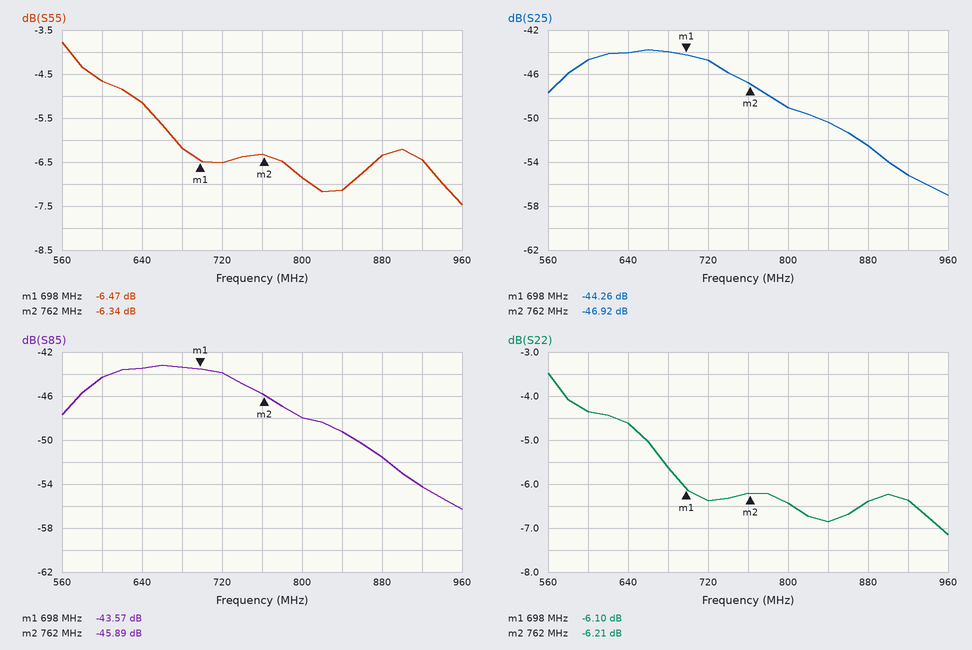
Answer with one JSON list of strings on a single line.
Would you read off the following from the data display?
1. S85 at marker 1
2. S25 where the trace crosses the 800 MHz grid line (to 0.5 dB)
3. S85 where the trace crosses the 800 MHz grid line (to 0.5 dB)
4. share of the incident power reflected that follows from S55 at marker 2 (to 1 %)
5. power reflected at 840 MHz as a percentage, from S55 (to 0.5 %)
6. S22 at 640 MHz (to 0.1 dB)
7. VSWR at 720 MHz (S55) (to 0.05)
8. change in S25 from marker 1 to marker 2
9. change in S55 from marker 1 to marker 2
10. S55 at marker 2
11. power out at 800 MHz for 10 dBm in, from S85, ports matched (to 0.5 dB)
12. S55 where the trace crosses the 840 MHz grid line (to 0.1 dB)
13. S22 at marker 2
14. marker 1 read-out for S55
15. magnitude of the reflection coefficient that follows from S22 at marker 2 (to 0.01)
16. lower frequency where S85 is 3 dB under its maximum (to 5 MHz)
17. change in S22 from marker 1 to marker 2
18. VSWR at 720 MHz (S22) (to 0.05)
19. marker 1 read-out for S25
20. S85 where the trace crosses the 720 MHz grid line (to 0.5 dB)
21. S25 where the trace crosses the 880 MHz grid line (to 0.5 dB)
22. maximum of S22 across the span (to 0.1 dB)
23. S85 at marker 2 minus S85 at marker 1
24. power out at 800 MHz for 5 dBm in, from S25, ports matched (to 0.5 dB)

["-43.57 dB", "-49.0 dB", "-48.0 dB", "23 %", "19.5 %", "-4.6 dB", "2.80", "-2.66 dB", "0.13 dB", "-6.34 dB", "-38.0 dBm", "-7.1 dB", "-6.21 dB", "-6.47 dB", "0.49", "575 MHz", "-0.11 dB", "2.85", "-44.26 dB", "-44.0 dB", "-52.5 dB", "-3.5 dB", "-2.32 dB", "-44.0 dBm"]
